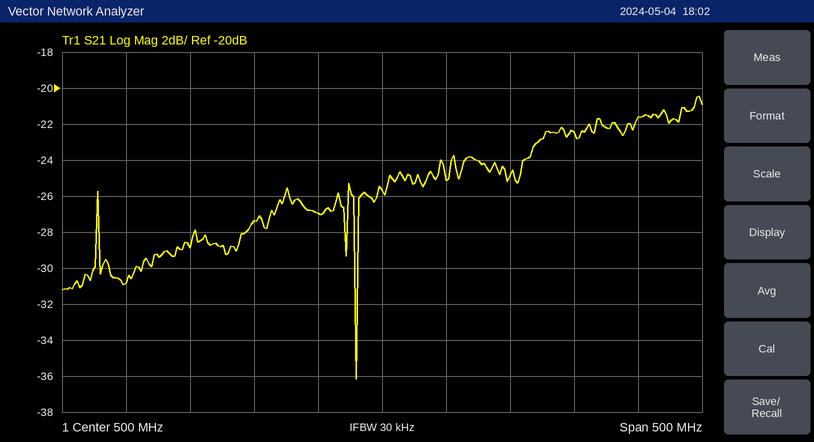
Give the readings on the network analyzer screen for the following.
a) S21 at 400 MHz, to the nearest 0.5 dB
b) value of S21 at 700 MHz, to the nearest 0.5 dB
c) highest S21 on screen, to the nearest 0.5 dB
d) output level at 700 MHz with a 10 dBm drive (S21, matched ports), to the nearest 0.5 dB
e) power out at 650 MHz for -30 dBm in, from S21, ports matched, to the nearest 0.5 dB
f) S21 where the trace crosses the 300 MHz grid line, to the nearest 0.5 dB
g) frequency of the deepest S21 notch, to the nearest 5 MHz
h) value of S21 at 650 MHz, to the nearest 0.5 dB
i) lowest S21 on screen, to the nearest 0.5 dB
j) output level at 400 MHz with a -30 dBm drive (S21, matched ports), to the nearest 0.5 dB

-27.5 dB
-21.5 dB
-20.5 dB
-11.5 dBm
-52.5 dBm
-31.0 dB
480 MHz
-22.5 dB
-36.0 dB
-57.5 dBm
